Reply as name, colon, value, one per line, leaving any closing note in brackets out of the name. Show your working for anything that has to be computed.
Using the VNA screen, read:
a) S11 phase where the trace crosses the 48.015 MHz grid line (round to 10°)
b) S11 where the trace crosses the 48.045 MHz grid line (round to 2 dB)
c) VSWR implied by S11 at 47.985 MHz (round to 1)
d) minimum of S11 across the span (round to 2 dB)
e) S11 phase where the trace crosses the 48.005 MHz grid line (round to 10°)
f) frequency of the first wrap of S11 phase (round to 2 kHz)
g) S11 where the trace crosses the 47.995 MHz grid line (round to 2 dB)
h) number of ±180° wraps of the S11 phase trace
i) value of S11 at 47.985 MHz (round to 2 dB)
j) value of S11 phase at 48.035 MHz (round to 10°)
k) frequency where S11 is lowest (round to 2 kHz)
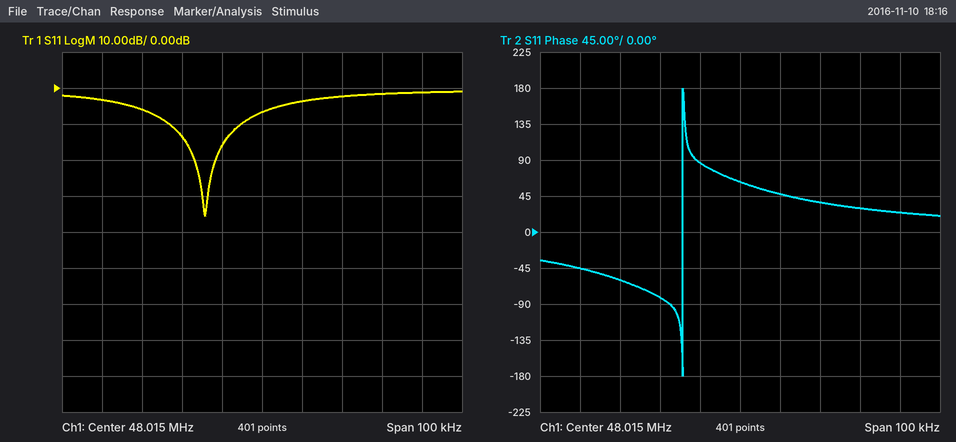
S11 phase where the trace crosses the 48.015 MHz grid line: 60°
S11 where the trace crosses the 48.045 MHz grid line: -2 dB
VSWR implied by S11 at 47.985 MHz: |Γ| = 10^(-6/20) = 0.5012; VSWR = (1 + 0.5012)/(1 − 0.5012) ≈ 3
minimum of S11 across the span: -36 dB
S11 phase where the trace crosses the 48.005 MHz grid line: 90°
frequency of the first wrap of S11 phase: 48.000 MHz
S11 where the trace crosses the 47.995 MHz grid line: -14 dB
number of ±180° wraps of the S11 phase trace: 1
value of S11 at 47.985 MHz: -6 dB
value of S11 phase at 48.035 MHz: 40°
frequency where S11 is lowest: 48.000 MHz
